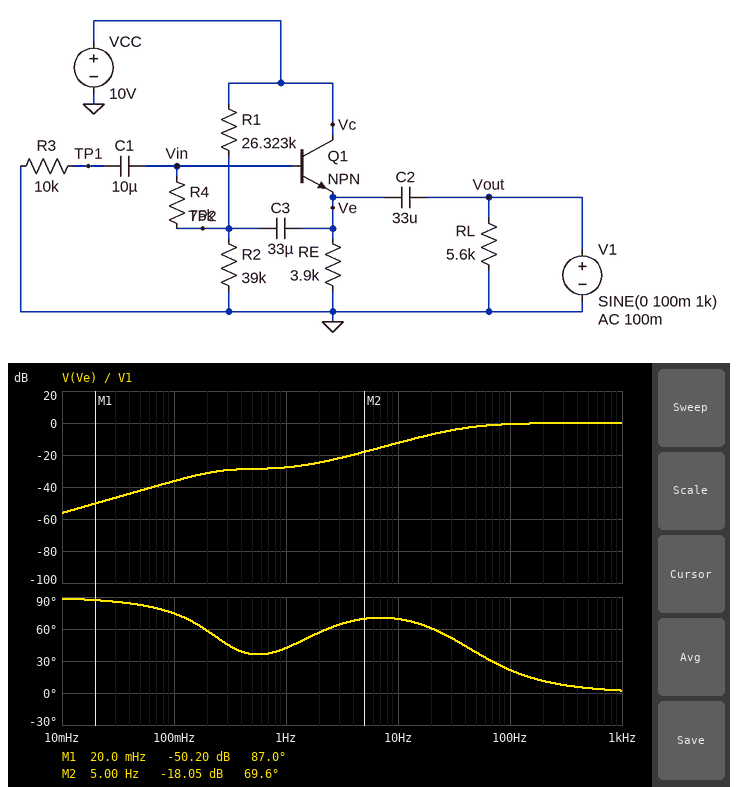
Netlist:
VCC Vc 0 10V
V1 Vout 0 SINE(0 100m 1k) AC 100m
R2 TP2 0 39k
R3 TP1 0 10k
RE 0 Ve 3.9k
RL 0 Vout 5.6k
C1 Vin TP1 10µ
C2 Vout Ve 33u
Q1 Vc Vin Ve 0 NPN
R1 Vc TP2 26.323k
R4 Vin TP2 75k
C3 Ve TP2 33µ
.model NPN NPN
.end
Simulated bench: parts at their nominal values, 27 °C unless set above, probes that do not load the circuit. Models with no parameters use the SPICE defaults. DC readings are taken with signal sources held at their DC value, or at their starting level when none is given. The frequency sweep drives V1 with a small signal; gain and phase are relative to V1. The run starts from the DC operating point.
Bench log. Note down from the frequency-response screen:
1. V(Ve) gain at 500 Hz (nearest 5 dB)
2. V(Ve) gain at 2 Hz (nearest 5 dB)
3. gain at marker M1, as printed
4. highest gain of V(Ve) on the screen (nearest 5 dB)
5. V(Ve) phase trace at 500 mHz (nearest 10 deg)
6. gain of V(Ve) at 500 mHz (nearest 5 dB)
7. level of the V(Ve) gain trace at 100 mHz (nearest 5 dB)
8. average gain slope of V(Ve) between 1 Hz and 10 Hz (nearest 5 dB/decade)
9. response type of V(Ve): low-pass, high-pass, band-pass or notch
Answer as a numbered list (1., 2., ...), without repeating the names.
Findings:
1. 0 dB
2. -25 dB
3. -50.20 dB
4. 0 dB
5. 40 deg
6. -30 dB
7. -35 dB
8. 15 dB/decade
9. high-pass
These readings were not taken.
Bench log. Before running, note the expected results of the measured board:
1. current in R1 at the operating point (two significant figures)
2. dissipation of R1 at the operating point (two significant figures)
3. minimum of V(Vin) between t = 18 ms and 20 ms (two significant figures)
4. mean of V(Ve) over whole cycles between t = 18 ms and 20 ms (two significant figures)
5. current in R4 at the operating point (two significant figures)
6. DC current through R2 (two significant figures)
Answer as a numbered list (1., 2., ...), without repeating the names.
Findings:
1. 160 µA
2. 670 µW
3. 4.9 V
4. 4.2 V
5. 11 µA
6. 150 µA
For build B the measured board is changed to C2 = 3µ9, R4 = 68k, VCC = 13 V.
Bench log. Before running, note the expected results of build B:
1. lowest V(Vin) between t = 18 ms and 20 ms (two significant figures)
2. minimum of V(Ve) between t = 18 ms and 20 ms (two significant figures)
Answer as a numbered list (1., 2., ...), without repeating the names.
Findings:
1. 6.5 V
2. 5.7 V
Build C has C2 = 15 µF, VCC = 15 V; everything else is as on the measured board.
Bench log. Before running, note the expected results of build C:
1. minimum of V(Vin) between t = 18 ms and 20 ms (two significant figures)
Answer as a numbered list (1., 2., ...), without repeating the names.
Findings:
1. 7.3 V
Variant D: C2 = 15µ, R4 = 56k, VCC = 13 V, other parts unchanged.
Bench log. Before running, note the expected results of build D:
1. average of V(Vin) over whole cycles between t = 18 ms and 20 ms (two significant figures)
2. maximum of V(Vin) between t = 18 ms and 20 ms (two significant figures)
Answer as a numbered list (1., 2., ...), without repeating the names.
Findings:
1. 6.7 V
2. 6.8 V
